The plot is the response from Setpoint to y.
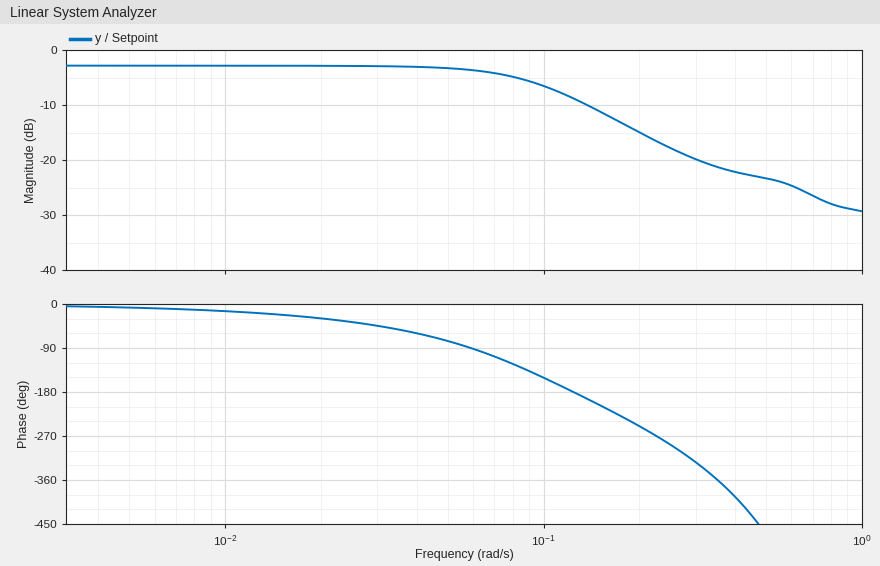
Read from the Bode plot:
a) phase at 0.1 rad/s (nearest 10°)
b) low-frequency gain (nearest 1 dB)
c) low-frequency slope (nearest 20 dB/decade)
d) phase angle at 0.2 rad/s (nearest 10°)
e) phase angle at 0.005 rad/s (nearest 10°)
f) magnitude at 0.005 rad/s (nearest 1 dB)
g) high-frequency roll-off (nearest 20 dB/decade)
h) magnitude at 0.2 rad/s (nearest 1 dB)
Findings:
-150°
-3 dB
0 dB/decade
-250°
-10°
-3 dB
-20 dB/decade
-15 dB
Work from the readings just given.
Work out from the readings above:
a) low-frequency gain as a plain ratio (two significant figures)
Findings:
0.71
